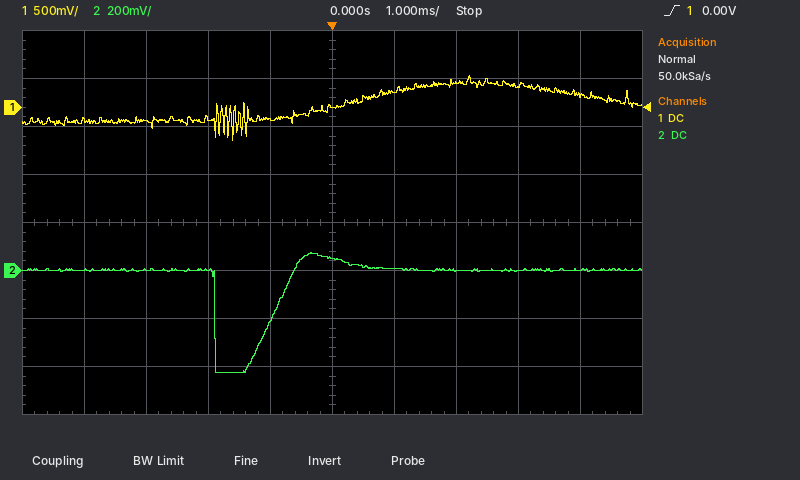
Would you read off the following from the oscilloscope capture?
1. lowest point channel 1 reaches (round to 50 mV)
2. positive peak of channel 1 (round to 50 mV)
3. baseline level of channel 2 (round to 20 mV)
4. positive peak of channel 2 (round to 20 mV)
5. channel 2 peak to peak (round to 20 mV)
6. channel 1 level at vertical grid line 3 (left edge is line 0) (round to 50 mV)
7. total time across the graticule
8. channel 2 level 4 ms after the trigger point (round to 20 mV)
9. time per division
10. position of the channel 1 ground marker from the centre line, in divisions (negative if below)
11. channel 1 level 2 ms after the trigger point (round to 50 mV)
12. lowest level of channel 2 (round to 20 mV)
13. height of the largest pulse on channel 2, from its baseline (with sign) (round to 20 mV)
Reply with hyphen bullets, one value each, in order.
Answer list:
- -350 mV
- 350 mV
- 0 mV
- 80 mV
- 500 mV
- -100 mV
- 10 ms
- 0 mV
- 1 ms
- +2.4 div
- 250 mV
- -420 mV
- -420 mV
